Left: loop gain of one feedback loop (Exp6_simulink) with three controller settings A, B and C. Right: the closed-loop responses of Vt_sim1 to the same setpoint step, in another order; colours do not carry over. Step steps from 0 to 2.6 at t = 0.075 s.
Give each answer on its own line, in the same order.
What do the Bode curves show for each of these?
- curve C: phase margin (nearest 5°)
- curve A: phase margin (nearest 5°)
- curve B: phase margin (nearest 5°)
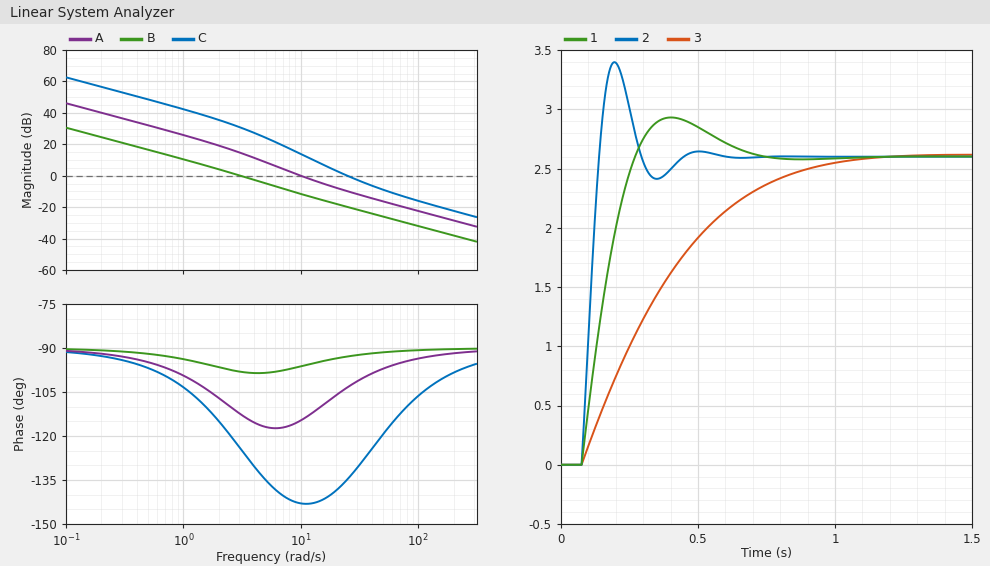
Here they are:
45°
65°
80°
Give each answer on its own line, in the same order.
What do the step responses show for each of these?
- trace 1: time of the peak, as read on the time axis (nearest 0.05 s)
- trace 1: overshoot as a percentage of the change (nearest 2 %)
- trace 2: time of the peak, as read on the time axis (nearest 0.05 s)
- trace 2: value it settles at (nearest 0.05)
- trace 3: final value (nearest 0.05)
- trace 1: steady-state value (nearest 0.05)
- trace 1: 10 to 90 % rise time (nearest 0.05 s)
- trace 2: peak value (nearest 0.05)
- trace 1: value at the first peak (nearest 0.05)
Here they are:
0.40 s
12 %
0.20 s
2.60
2.60
2.60
0.15 s
3.40
2.95
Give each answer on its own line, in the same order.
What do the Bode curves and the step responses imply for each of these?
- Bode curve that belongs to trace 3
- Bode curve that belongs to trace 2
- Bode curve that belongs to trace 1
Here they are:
B
C
A
